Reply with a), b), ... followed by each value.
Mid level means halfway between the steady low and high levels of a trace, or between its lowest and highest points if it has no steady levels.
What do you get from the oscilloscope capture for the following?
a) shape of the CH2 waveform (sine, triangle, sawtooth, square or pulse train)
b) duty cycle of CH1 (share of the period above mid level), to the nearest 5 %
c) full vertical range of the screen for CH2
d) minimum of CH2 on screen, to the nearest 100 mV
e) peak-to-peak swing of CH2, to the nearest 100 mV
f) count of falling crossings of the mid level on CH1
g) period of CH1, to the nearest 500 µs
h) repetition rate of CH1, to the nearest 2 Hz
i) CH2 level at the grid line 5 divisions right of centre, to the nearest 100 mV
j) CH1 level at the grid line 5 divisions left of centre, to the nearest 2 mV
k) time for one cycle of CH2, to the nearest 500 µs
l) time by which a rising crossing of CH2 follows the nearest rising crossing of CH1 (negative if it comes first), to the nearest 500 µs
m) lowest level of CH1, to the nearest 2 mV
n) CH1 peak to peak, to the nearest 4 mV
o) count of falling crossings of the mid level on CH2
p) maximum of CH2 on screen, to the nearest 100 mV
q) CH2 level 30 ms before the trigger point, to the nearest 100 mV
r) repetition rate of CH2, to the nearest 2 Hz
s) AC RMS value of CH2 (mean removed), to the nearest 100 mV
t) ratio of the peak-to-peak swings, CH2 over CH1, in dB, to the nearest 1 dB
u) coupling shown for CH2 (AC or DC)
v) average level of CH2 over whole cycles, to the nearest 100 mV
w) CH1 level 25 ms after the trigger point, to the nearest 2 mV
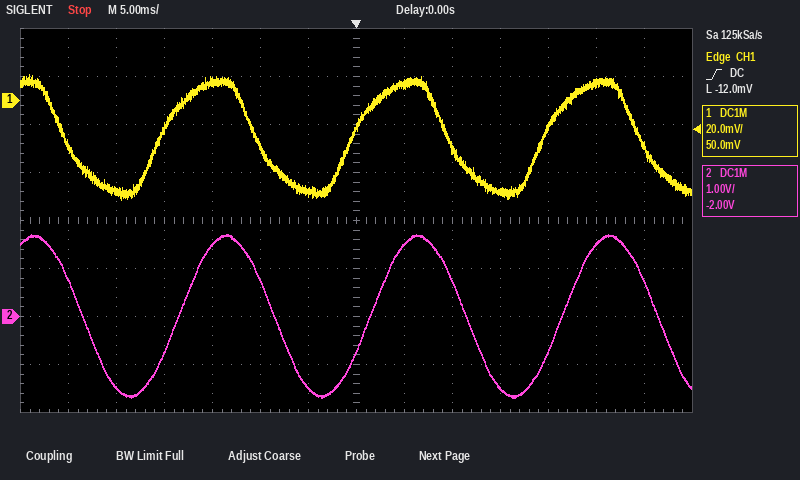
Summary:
a) sine
b) 50 %
c) 8 V
d) -1.7 V
e) 3.4 V
f) 4
g) 20.0 ms
h) 50 Hz
i) 1.5 V
j) -38 mV
k) 20.0 ms
l) +2.0 ms
m) -42 mV
n) 52 mV
o) 4
p) 1.7 V
q) 800 mV
r) 50 Hz
s) 1.2 V
t) 36 dB
u) DC
v) 0.0 V
w) 8 mV
